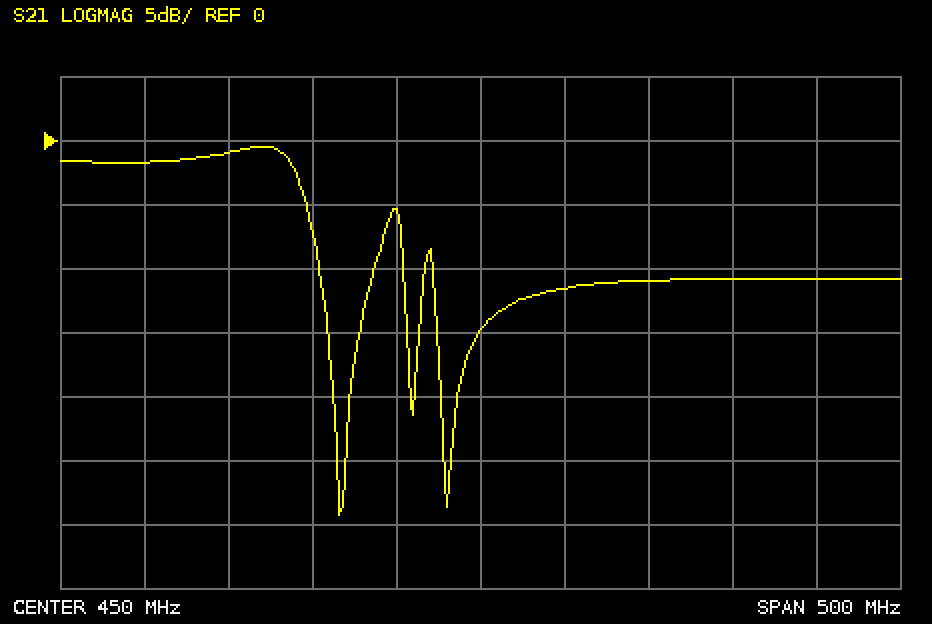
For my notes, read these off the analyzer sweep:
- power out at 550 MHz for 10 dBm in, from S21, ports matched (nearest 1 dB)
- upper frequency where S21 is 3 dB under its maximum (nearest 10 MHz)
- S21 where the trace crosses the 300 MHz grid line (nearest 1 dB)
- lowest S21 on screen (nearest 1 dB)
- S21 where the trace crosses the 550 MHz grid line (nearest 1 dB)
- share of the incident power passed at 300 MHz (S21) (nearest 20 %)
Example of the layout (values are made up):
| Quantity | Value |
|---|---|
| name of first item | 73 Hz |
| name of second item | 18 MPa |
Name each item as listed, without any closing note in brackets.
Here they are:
| Quantity | Value |
|---|---|
| power out at 550 MHz for 10 dBm in, from S21, ports matched | -1 dBm |
| upper frequency where S21 is 3 dB under its maximum | 340 MHz |
| S21 where the trace crosses the 300 MHz grid line | -1 dB |
| lowest S21 on screen | -29 dB |
| S21 where the trace crosses the 550 MHz grid line | -11 dB |
| share of the incident power passed at 300 MHz (S21) | 80 % |
